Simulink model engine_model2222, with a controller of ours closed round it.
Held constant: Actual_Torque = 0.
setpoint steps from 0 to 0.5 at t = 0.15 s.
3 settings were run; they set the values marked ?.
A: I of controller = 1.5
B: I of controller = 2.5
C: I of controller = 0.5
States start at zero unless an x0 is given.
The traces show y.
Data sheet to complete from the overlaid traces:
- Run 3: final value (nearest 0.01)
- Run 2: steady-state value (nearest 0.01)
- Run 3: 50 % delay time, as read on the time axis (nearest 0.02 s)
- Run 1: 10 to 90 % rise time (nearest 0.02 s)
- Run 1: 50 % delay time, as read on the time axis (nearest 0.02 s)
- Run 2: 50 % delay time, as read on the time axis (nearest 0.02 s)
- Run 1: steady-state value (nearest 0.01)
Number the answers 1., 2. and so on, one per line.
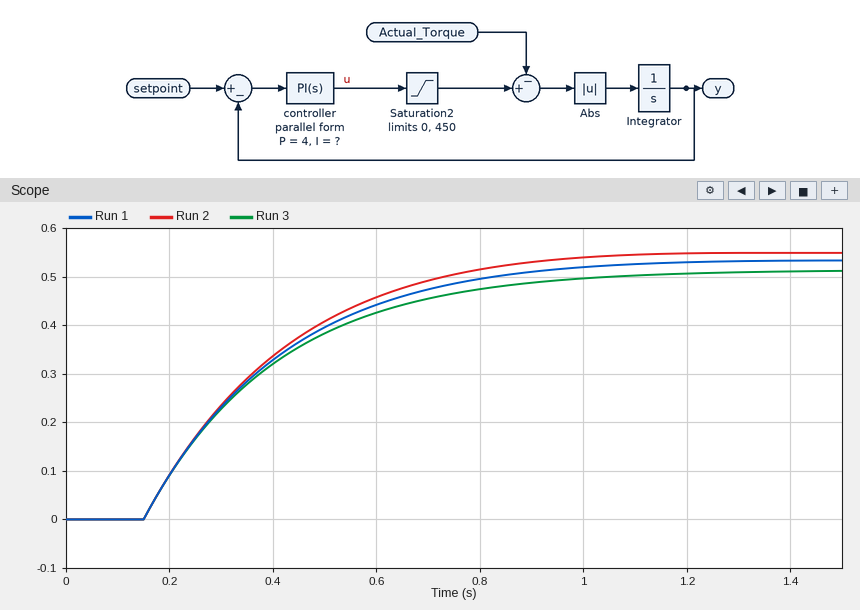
1. 0.51
2. 0.55
3. 0.32 s
4. 0.54 s
5. 0.34 s
6. 0.34 s
7. 0.53
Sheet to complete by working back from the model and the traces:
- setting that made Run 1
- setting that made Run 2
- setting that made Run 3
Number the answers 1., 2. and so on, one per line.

1. A
2. B
3. C
